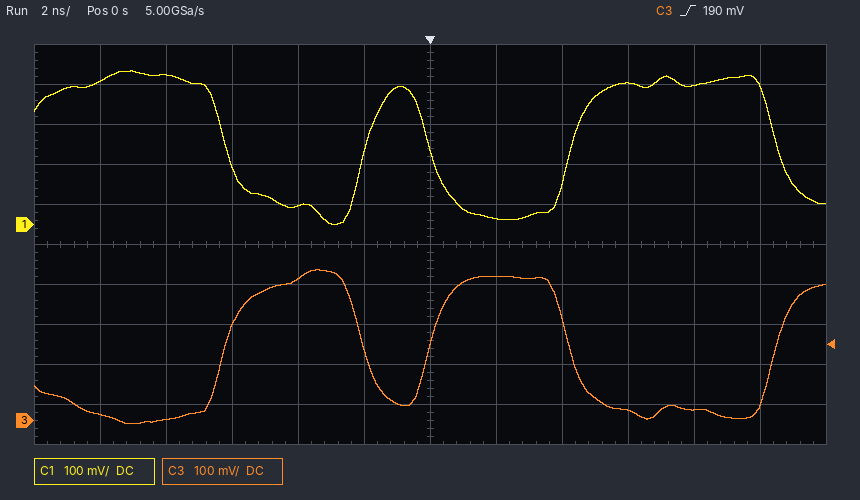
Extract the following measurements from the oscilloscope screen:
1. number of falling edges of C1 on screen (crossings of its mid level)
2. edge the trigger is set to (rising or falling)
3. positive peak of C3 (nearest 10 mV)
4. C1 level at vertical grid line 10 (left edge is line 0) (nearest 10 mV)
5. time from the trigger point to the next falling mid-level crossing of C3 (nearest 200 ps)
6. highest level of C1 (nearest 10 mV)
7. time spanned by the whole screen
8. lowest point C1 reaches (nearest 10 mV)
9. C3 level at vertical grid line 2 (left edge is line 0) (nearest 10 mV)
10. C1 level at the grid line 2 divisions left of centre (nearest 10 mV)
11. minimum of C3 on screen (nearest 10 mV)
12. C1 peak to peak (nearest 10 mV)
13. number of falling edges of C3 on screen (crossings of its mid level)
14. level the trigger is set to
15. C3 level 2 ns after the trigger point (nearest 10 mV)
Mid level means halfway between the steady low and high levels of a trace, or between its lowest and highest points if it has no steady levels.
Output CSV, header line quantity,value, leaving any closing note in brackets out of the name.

quantity,value
number of falling edges of C1 on screen,3
edge the trigger is set to,rising
positive peak of C3,380 mV
C1 level at vertical grid line 10 (left edge is line 0),350 mV
time from the trigger point to the next falling mid-level crossing of C3,4.2 ns
highest level of C1,380 mV
time spanned by the whole screen,24 ns
lowest point C1 reaches,0 mV
C3 level at vertical grid line 2 (left edge is line 0),0 mV
C1 level at the grid line 2 divisions left of centre,50 mV
minimum of C3 on screen,-10 mV
C1 peak to peak,380 mV
number of falling edges of C3 on screen,2
level the trigger is set to,190 mV
C3 level 2 ns after the trigger point,360 mV
